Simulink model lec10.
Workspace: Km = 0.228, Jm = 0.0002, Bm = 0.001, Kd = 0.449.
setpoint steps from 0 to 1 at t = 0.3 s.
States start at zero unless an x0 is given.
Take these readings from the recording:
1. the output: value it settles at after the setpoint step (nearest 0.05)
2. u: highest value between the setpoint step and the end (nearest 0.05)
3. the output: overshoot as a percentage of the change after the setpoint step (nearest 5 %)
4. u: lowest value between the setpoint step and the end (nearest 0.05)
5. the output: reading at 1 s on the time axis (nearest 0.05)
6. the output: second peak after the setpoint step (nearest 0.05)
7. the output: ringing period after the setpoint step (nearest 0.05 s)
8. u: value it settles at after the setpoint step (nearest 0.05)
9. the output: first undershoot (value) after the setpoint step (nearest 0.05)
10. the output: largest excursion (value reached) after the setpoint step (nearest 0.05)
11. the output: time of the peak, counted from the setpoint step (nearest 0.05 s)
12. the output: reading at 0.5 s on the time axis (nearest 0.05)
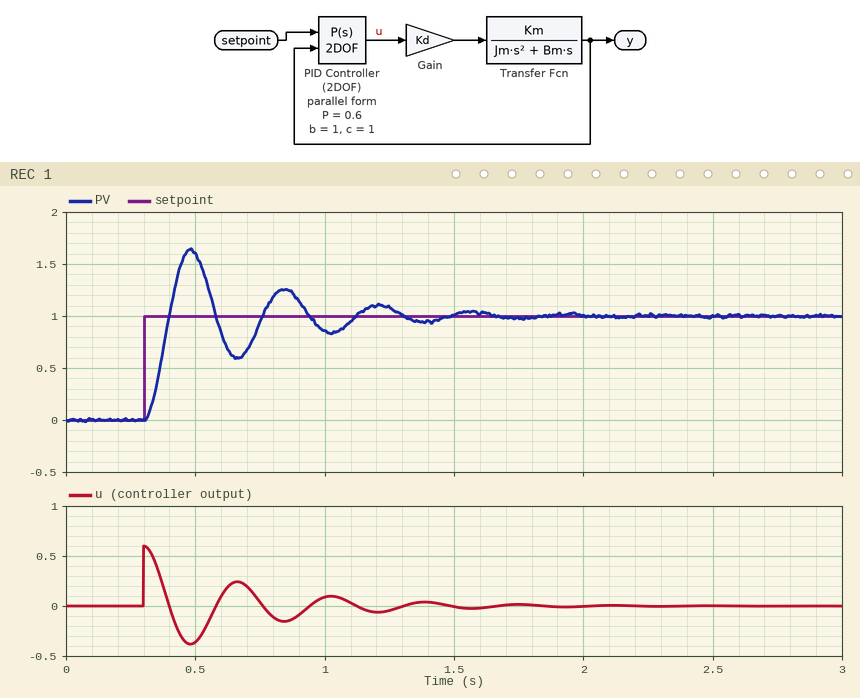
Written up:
1.00
0.60
65 %
-0.40
0.85
1.25
0.35 s
0.00
0.60
1.65
0.20 s
1.60
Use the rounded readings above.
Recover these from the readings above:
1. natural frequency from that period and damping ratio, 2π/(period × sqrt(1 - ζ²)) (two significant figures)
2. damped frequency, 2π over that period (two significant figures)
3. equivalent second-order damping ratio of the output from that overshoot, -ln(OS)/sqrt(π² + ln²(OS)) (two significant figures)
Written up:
18 rad/s
18 rad/s
0.14
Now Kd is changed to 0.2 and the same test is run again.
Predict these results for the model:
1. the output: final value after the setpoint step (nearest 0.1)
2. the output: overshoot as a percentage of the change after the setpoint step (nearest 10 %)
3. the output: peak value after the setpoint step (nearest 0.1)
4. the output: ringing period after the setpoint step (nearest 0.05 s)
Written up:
1.0
50 %
1.5
0.55 s
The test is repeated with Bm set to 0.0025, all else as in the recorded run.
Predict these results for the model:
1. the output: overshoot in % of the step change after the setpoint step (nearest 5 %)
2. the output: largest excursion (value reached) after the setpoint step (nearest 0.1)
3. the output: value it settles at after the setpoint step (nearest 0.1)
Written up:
30 %
1.3
1.0
